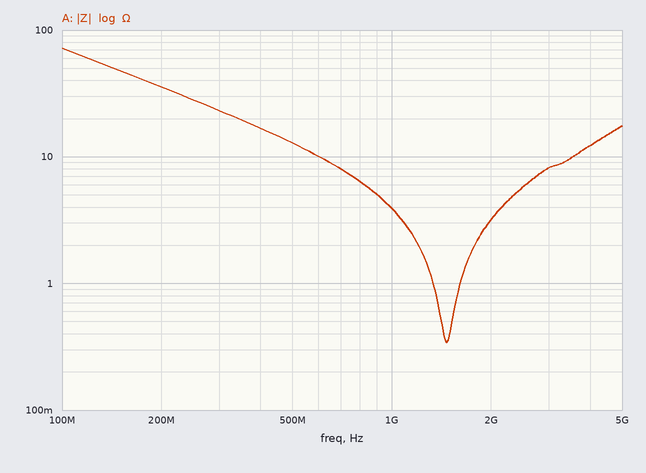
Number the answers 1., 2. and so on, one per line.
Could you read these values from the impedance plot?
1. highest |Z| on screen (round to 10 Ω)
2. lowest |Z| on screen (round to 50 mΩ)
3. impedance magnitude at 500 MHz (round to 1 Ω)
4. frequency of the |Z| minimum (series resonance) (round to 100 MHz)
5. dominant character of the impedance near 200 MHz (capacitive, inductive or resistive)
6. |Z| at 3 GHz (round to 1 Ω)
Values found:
1. 70 Ω
2. 350 mΩ
3. 13 Ω
4. 1.5 GHz
5. capacitive
6. 8 Ω
